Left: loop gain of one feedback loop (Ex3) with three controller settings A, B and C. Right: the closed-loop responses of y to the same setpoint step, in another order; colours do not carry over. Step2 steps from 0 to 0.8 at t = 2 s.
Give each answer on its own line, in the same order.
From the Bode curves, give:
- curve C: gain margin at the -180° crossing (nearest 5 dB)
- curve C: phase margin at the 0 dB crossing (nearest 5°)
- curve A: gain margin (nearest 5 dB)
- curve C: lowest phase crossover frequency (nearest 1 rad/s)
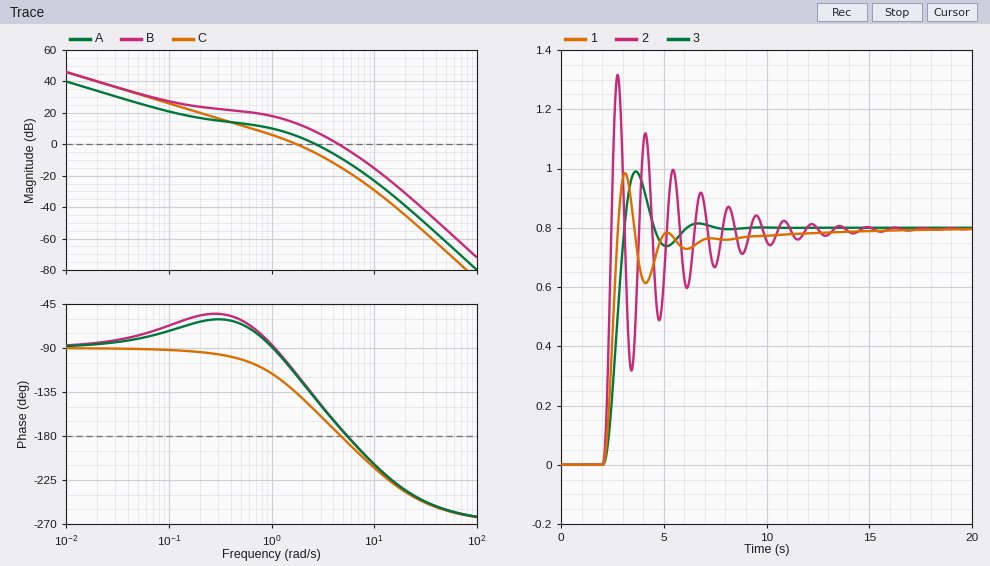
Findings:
15 dB
45°
10 dB
5 rad/s
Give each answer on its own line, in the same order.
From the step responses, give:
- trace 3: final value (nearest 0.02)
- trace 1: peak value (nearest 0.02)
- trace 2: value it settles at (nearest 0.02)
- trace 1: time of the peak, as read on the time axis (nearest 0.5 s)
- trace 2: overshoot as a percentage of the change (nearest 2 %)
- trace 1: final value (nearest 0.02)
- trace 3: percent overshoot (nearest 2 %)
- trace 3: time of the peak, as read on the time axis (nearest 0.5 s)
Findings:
0.80
0.98
0.80
3.0 s
64 %
0.80
24 %
3.5 s
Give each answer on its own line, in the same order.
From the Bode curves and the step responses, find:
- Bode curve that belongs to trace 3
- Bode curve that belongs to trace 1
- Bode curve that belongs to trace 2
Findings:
C
A
B
